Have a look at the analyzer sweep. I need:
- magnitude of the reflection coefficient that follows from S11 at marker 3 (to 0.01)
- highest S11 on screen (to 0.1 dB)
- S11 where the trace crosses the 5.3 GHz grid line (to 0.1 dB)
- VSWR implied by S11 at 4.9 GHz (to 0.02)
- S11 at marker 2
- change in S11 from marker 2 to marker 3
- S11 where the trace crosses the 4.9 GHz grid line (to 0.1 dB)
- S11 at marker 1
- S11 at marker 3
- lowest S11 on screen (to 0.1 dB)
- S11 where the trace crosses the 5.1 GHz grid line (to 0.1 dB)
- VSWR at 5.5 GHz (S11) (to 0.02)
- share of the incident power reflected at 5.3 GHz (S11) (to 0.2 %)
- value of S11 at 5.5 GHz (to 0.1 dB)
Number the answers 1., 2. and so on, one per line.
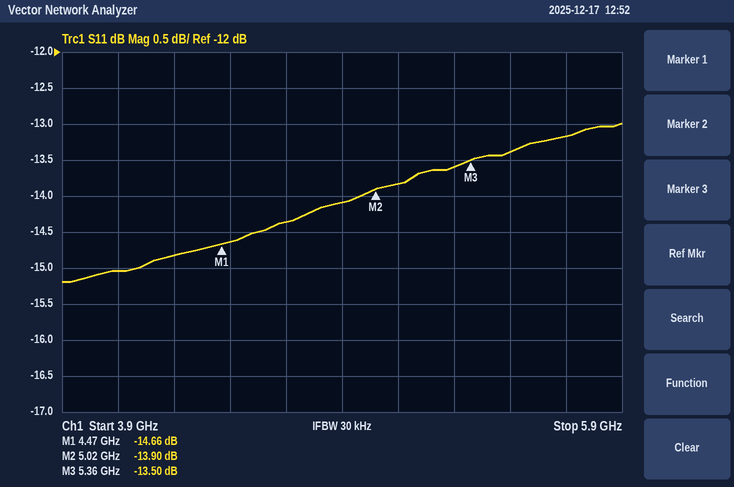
1. 0.21
2. -13.0 dB
3. -13.6 dB
4. 1.50
5. -13.90 dB
6. 0.40 dB
7. -14.1 dB
8. -14.66 dB
9. -13.50 dB
10. -15.2 dB
11. -13.8 dB
12. 1.54
13. 4.4 %
14. -13.4 dB
